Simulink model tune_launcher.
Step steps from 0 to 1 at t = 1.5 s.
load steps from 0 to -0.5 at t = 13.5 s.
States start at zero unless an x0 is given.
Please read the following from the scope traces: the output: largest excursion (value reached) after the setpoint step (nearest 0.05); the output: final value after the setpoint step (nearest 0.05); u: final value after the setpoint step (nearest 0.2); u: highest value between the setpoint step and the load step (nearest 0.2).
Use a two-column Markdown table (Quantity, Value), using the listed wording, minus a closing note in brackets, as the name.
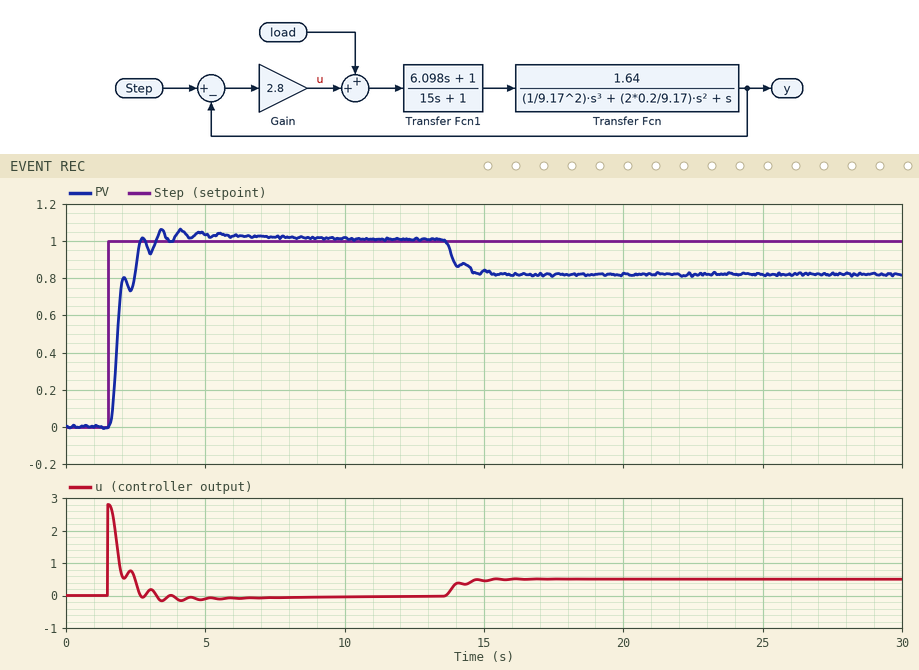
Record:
| Quantity | Value |
|---|---|
| the output: largest excursion (value reached) after the setpoint step | 1.05 |
| the output: final value after the setpoint step | 1.00 |
| u: final value after the setpoint step | 0.0 |
| u: highest value between the setpoint step and the load step | 2.8 |
